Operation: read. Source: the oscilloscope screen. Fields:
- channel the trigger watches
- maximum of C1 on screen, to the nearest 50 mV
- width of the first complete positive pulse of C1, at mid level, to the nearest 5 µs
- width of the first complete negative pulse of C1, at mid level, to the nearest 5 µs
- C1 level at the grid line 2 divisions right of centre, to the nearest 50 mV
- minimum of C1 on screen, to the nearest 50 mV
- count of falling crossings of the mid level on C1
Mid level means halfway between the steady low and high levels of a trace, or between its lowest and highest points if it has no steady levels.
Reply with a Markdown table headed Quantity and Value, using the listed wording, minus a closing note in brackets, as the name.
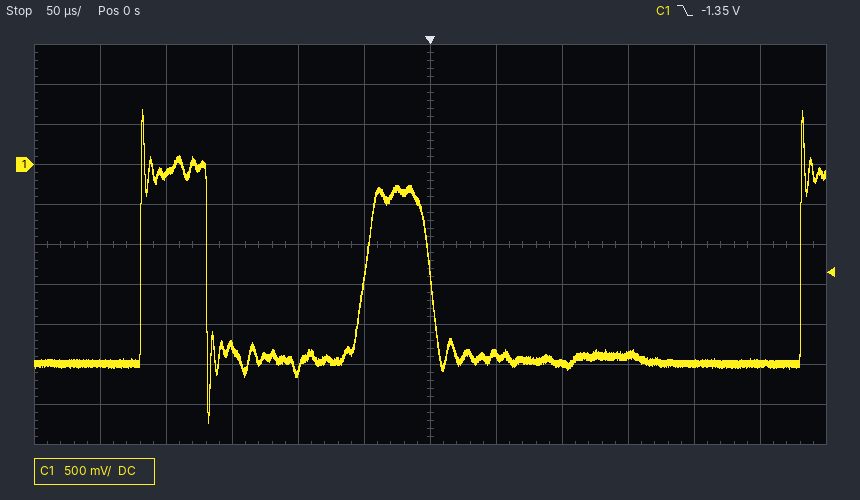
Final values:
| Quantity | Value |
|---|---|
| channel the trigger watches | C1 |
| maximum of C1 on screen, to the nearest 50 mV | 700 mV |
| width of the first complete positive pulse of C1, at mid level, to the nearest 5 µs | 50 µs |
| width of the first complete negative pulse of C1, at mid level, to the nearest 5 µs | 120 µs |
| C1 level at the grid line 2 divisions right of centre, to the nearest 50 mV | -2.50 V |
| minimum of C1 on screen, to the nearest 50 mV | -3.25 V |
| count of falling crossings of the mid level on C1 | 2 |
